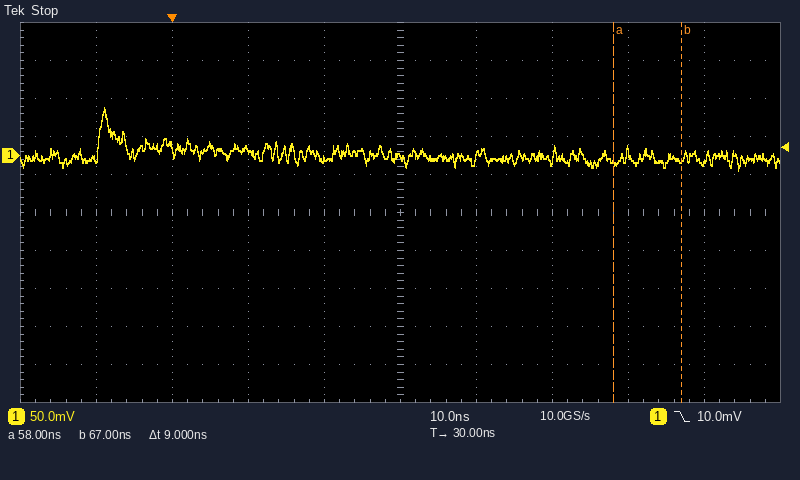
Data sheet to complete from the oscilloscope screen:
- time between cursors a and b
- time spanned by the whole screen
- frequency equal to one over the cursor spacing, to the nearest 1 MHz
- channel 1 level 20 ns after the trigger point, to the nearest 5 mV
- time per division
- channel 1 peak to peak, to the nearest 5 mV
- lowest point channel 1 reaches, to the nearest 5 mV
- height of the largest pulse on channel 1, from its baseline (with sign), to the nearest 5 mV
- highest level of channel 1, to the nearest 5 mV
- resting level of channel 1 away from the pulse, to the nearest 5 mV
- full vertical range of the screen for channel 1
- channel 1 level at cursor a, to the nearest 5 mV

9 ns
100 ns
111 MHz
-5 mV
10 ns
85 mV
-20 mV
+65 mV
65 mV
0 mV
500 mV
-10 mV
